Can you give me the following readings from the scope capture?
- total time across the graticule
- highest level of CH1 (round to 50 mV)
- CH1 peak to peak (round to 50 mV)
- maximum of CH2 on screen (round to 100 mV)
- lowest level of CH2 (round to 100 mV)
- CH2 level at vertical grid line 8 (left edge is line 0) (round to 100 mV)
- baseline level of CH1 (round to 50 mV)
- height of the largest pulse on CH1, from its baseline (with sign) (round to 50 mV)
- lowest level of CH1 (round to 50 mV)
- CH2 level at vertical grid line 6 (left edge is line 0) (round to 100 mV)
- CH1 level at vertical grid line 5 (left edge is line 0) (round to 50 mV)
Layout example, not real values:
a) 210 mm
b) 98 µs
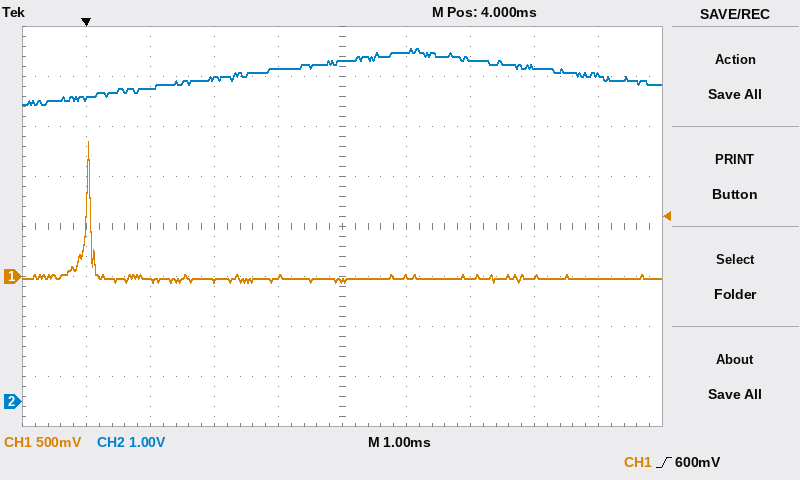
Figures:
a) 10 ms
b) 1.35 V
c) 1.40 V
d) 7.1 V
e) 5.9 V
f) 6.7 V
g) 0 mV
h) +1.35 V
i) -50 mV
j) 7.0 V
k) -50 mV
